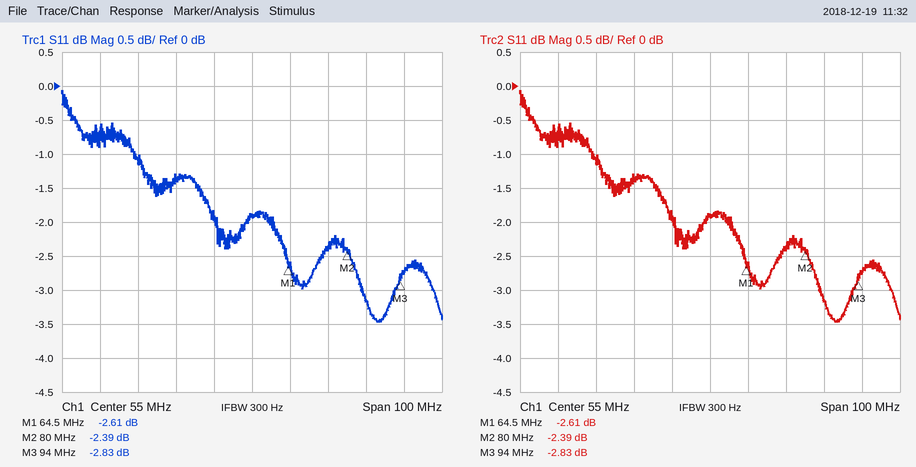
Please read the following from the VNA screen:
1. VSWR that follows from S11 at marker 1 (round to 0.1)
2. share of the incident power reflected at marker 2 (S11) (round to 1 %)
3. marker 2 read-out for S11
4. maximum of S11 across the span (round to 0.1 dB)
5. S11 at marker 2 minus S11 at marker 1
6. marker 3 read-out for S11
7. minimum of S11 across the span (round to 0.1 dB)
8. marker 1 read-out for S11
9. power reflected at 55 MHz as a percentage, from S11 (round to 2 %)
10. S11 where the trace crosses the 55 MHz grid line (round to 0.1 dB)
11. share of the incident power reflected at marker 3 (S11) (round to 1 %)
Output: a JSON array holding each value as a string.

["6.7", "58 %", "-2.39 dB", "-0.1 dB", "0.22 dB", "-2.83 dB", "-3.5 dB", "-2.61 dB", "64 %", "-1.9 dB", "52 %"]
